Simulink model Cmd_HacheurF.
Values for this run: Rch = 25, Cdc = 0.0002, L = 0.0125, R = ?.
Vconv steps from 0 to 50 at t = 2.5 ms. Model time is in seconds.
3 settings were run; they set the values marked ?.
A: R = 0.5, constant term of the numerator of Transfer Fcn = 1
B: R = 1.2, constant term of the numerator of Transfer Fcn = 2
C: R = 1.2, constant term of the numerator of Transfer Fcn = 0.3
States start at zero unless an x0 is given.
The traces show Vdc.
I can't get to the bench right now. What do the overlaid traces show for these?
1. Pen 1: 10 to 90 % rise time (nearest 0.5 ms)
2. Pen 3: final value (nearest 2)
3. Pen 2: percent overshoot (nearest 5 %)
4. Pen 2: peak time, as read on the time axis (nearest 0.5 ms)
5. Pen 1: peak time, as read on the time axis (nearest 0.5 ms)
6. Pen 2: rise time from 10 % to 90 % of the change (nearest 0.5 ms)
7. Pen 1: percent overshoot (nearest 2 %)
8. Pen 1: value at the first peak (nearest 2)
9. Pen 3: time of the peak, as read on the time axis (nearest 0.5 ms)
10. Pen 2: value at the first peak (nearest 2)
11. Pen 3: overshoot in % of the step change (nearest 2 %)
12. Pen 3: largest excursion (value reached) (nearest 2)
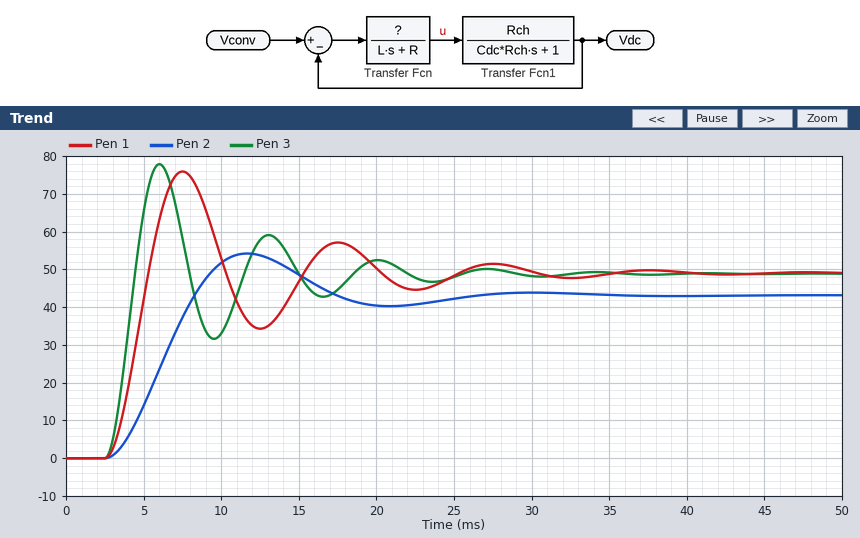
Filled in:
2.0 ms
48
25 %
11.5 ms
7.5 ms
4.0 ms
54 %
76
6.0 ms
54
60 %
78
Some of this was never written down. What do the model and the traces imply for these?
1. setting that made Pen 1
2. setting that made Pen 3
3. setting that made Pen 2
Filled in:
A
B
C
